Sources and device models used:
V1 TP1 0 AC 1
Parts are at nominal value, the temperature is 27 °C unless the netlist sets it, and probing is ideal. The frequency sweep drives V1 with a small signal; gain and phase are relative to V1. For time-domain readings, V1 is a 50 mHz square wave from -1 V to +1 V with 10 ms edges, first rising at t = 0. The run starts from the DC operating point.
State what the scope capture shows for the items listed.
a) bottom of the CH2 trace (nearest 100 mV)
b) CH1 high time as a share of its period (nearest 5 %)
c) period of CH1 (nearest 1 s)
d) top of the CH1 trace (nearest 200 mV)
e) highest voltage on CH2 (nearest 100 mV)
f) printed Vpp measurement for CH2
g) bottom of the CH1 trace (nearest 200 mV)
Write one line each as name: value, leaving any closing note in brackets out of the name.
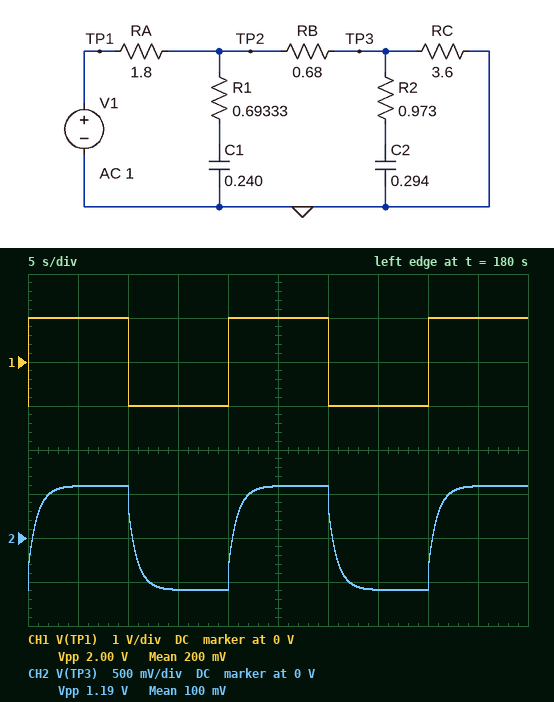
bottom of the CH2 trace: -600 mV
CH1 high time as a share of its period: 50 %
period of CH1: 20 s
top of the CH1 trace: 1.0 V
highest voltage on CH2: 600 mV
printed Vpp measurement for CH2: 1.19 V
bottom of the CH1 trace: -1.0 V
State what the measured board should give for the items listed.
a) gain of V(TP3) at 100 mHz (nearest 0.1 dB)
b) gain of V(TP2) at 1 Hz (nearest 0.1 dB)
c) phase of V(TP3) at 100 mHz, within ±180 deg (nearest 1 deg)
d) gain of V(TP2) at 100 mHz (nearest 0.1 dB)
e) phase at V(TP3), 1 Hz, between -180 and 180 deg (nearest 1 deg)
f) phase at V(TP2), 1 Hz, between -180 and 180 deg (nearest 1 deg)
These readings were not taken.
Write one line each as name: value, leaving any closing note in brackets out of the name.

gain of V(TP3) at 100 mHz: -5.7 dB
gain of V(TP2) at 1 Hz: -11.7 dB
phase of V(TP3) at 100 mHz, within ±180 deg: -24 deg
gain of V(TP2) at 100 mHz: -4.0 dB
phase at V(TP3), 1 Hz, between -180 and 180 deg: -34 deg
phase at V(TP2), 1 Hz, between -180 and 180 deg: -24 deg
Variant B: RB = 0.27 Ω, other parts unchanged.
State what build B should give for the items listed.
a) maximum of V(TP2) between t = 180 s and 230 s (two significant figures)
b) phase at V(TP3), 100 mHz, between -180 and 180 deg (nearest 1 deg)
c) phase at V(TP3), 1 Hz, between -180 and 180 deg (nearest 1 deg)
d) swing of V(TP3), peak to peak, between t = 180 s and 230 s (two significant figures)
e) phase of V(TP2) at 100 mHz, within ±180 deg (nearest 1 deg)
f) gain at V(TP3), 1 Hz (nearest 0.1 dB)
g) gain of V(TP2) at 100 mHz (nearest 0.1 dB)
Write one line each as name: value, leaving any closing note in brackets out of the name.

maximum of V(TP2) between t = 180 s and 230 s: 680 mV
phase at V(TP3), 100 mHz, between -180 and 180 deg: -22 deg
phase at V(TP3), 1 Hz, between -180 and 180 deg: -30 deg
swing of V(TP3), peak to peak, between t = 180 s and 230 s: 1.3 V
phase of V(TP2) at 100 mHz, within ±180 deg: -19 deg
gain at V(TP3), 1 Hz: -14.8 dB
gain of V(TP2) at 100 mHz: -4.3 dB
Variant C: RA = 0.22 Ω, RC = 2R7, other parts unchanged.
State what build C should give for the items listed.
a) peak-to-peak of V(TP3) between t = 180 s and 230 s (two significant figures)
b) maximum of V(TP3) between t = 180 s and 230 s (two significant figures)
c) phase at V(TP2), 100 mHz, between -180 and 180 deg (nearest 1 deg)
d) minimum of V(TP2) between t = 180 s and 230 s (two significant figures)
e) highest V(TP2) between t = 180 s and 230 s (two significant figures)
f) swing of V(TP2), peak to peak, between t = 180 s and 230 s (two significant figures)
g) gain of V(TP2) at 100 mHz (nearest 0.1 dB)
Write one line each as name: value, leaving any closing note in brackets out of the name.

peak-to-peak of V(TP3) between t = 180 s and 230 s: 1.5 V
maximum of V(TP3) between t = 180 s and 230 s: 750 mV
phase at V(TP2), 100 mHz, between -180 and 180 deg: -3 deg
minimum of V(TP2) between t = 180 s and 230 s: -940 mV
highest V(TP2) between t = 180 s and 230 s: 940 mV
swing of V(TP2), peak to peak, between t = 180 s and 230 s: 1.9 V
gain of V(TP2) at 100 mHz: -0.6 dB
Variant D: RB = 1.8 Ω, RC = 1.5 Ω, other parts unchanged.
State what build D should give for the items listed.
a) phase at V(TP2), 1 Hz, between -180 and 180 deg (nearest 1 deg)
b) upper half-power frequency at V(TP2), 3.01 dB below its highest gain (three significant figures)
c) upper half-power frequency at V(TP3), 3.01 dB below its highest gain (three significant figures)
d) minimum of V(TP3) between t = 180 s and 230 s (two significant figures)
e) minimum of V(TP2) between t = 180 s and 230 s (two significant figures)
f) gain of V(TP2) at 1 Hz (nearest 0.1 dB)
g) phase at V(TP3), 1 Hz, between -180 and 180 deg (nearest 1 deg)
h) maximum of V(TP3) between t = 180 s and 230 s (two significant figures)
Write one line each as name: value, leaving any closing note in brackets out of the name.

phase at V(TP2), 1 Hz, between -180 and 180 deg: -24 deg
upper half-power frequency at V(TP2), 3.01 dB below its highest gain: 351 mHz
upper half-power frequency at V(TP3), 3.01 dB below its highest gain: 227 mHz
minimum of V(TP3) between t = 180 s and 230 s: -290 mV
minimum of V(TP2) between t = 180 s and 230 s: -650 mV
gain of V(TP2) at 1 Hz: -10.6 dB
phase at V(TP3), 1 Hz, between -180 and 180 deg: -36 deg
maximum of V(TP3) between t = 180 s and 230 s: 290 mV
